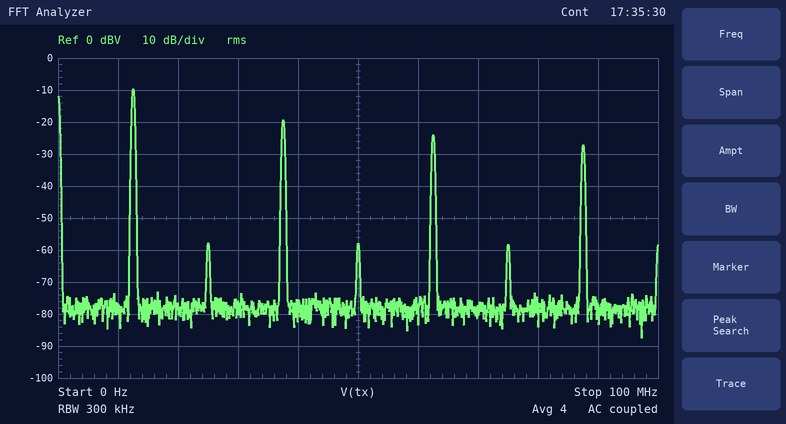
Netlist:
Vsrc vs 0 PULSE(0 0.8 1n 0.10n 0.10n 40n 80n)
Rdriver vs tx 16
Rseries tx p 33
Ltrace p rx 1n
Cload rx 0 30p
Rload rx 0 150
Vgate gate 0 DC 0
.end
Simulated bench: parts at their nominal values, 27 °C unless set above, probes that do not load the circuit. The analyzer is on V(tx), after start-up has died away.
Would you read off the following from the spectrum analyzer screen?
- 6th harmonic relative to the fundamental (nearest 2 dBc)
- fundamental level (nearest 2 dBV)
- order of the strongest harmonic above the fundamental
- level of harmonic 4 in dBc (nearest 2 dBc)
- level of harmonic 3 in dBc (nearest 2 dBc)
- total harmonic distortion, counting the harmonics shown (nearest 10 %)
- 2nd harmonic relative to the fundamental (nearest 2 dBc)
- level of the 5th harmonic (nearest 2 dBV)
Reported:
-48 dBc
-10 dBV
3
-48 dBc
-10 dBc
40 %
-48 dBc
-24 dBV
